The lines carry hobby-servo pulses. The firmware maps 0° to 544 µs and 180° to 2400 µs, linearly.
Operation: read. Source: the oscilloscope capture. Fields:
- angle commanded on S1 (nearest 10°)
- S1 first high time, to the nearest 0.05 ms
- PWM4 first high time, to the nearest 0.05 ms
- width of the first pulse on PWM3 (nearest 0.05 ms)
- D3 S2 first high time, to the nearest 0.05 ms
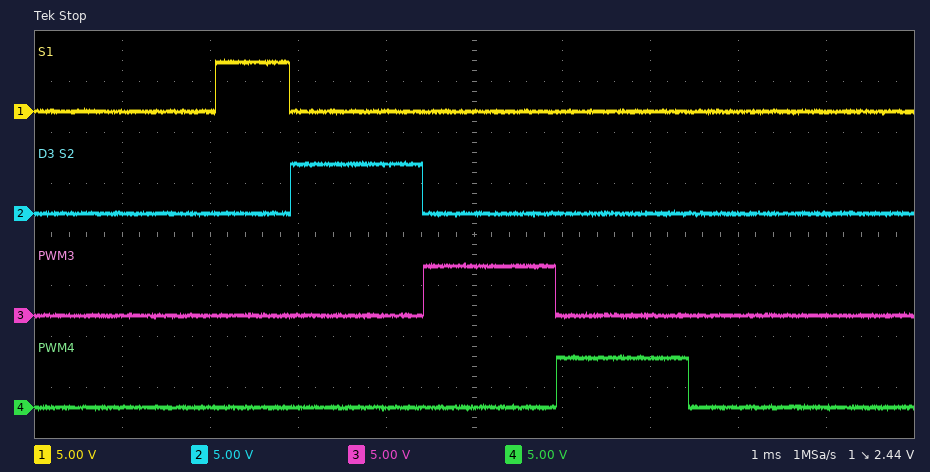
30°
0.85 ms
1.50 ms
1.50 ms
1.50 ms
